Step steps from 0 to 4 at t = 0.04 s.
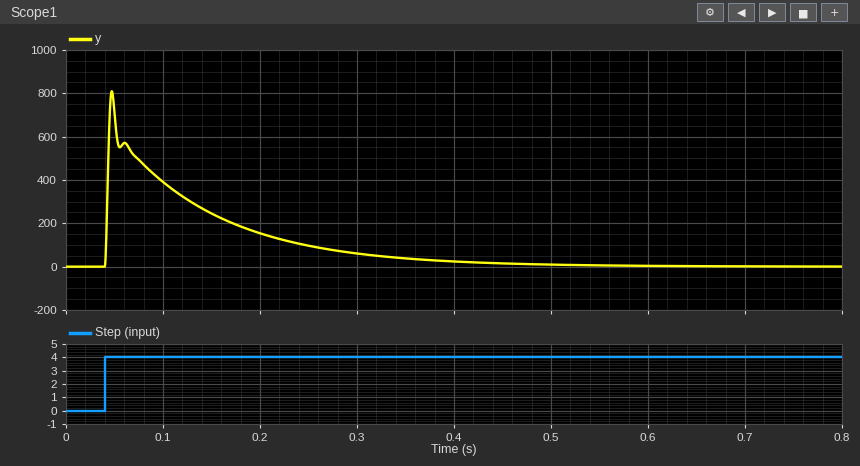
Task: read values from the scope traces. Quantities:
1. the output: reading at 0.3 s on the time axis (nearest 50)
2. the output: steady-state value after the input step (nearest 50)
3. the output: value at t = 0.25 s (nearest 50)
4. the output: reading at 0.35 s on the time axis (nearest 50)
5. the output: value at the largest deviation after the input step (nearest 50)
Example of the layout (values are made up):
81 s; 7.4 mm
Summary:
50; 0; 100; 50; 800
